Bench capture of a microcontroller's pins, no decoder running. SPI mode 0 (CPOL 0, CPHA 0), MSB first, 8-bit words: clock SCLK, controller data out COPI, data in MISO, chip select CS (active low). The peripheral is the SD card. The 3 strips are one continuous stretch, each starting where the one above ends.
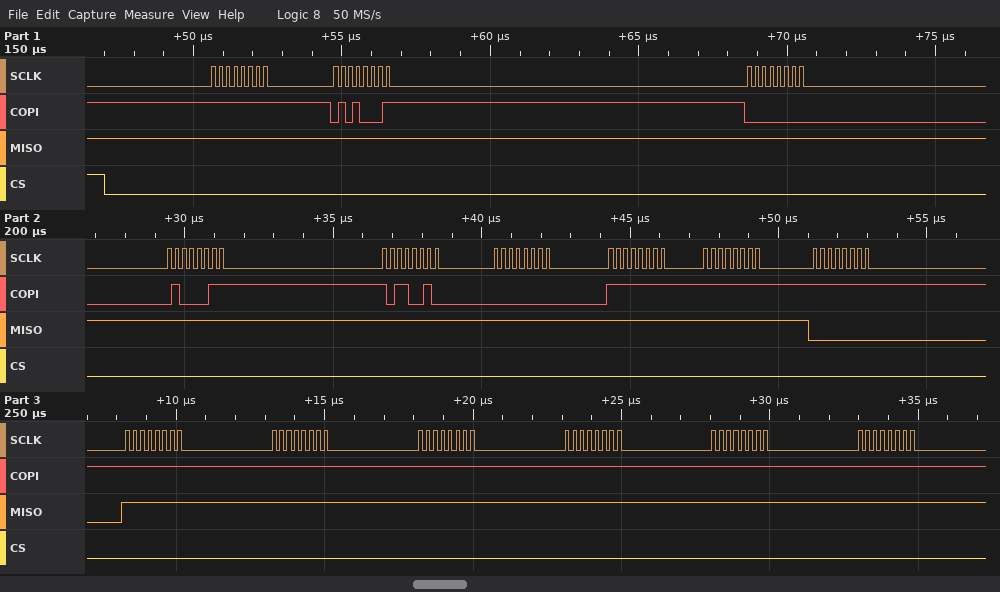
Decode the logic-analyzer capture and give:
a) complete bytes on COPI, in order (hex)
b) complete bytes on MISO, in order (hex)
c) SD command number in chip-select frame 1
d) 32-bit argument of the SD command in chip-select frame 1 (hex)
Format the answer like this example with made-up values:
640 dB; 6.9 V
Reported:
0xFF 0x51 0x00 0x43 0xB2 0x00 0xFF 0xFF 0xFF 0xFF 0xFF 0xFF 0xFF 0xFF 0xFF; 0xFF 0xFF 0xFF 0xFF 0xFF 0xFF 0xFF 0xFF 0x00 0xFF 0xFF 0xFF 0xFF 0xFF 0xFF; CMD17; 0x0043B200
